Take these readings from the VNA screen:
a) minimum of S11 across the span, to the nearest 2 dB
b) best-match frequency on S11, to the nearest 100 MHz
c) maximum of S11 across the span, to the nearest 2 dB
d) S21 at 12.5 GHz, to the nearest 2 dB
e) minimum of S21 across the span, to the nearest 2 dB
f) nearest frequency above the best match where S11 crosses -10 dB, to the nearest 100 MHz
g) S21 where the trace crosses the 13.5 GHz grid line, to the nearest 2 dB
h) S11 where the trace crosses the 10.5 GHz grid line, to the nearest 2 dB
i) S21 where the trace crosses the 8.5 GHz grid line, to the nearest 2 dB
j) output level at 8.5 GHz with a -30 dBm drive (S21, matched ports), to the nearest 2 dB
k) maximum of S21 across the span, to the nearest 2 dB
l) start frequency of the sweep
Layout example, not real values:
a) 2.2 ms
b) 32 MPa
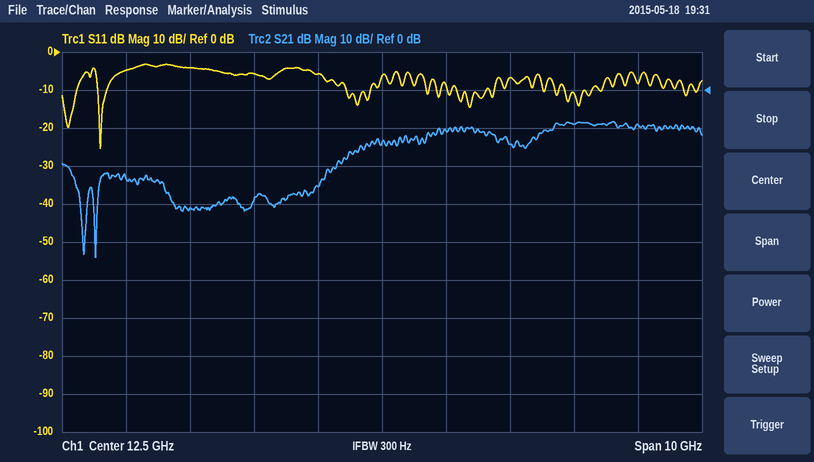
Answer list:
a) -26 dB
b) 8.1 GHz
c) -4 dB
d) -14 dB
e) -44 dB
f) 8.2 GHz
g) -10 dB
h) -6 dB
i) -24 dB
j) -54 dBm
k) -8 dB
l) 7.5 GHz
